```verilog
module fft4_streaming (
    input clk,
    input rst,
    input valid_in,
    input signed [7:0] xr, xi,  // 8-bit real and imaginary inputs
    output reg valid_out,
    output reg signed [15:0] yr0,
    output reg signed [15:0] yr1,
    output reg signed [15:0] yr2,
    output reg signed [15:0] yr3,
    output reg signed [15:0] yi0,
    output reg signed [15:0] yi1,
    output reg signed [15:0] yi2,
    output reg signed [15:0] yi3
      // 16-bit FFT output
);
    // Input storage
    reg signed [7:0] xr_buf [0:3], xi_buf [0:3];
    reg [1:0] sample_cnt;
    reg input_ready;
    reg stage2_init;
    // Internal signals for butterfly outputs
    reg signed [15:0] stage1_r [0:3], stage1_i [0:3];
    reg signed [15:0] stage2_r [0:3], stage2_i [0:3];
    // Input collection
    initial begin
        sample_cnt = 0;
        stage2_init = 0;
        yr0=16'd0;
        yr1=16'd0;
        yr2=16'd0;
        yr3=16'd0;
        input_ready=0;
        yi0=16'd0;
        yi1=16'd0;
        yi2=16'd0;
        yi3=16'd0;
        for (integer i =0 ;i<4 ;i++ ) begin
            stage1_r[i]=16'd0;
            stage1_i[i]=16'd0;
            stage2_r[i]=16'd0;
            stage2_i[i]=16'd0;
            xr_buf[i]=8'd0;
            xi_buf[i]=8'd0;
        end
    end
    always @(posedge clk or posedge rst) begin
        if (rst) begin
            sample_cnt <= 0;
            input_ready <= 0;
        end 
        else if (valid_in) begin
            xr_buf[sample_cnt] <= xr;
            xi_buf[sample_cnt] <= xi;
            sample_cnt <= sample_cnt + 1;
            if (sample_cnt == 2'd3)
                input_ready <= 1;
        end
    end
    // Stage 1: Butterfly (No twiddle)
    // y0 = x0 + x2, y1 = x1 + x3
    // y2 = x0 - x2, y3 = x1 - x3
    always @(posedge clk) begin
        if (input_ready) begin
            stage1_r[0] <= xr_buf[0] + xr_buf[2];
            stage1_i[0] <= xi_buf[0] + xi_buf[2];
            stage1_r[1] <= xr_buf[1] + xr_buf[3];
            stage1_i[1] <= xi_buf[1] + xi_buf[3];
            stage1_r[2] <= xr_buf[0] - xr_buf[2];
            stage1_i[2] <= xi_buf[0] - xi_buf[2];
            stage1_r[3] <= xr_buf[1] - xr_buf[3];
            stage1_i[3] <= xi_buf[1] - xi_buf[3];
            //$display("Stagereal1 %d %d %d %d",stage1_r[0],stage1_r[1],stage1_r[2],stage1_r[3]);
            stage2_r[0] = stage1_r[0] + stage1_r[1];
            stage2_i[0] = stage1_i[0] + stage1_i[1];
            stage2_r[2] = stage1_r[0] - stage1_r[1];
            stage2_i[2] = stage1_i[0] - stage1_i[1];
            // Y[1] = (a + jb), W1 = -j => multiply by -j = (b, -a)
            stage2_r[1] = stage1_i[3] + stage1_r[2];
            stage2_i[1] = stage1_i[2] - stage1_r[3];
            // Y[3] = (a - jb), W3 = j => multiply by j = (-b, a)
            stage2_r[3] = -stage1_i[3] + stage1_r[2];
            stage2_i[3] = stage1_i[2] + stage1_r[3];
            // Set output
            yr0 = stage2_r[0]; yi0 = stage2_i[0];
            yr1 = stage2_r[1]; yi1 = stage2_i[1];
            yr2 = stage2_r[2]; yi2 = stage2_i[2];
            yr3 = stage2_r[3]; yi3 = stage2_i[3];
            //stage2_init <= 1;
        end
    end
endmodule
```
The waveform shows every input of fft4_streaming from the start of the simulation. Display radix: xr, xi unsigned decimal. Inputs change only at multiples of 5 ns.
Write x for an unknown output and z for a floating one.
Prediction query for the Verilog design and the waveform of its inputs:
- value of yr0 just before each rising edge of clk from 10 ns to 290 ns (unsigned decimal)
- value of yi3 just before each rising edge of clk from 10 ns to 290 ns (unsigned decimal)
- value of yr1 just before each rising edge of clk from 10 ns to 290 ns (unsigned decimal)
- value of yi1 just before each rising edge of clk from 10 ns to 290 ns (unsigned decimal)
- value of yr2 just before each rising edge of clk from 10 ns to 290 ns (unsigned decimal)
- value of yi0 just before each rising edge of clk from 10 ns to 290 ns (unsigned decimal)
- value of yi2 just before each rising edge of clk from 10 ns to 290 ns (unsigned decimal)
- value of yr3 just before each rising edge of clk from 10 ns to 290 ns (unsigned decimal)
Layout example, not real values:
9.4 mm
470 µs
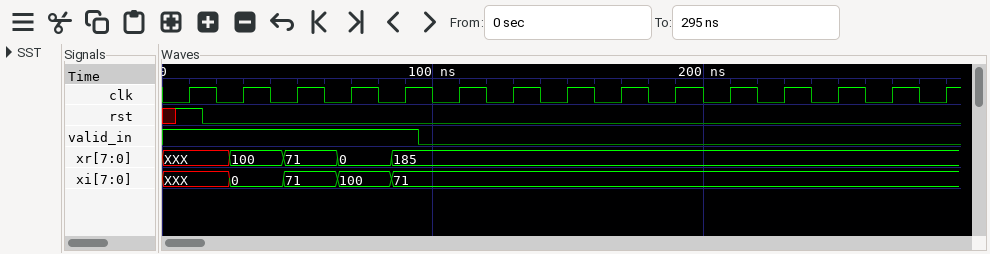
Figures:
0, 0, 0, 0, 0, 0, 0, 100, 100, 100, 100, 100, 100, 100, 100
0, 0, 0, 0, 0, 0, 0, 42, 42, 42, 42, 42, 42, 42, 42
0, 0, 0, 0, 0, 0, 0, 100, 100, 100, 100, 100, 100, 100, 100
0, 0, 0, 0, 0, 0, 0, 65294, 65294, 65294, 65294, 65294, 65294, 65294, 65294
0, 0, 0, 0, 0, 0, 0, 100, 100, 100, 100, 100, 100, 100, 100
0, 0, 0, 0, 0, 0, 0, 242, 242, 242, 242, 242, 242, 242, 242
0, 0, 0, 0, 0, 0, 0, 65494, 65494, 65494, 65494, 65494, 65494, 65494, 65494
0, 0, 0, 0, 0, 0, 0, 100, 100, 100, 100, 100, 100, 100, 100
